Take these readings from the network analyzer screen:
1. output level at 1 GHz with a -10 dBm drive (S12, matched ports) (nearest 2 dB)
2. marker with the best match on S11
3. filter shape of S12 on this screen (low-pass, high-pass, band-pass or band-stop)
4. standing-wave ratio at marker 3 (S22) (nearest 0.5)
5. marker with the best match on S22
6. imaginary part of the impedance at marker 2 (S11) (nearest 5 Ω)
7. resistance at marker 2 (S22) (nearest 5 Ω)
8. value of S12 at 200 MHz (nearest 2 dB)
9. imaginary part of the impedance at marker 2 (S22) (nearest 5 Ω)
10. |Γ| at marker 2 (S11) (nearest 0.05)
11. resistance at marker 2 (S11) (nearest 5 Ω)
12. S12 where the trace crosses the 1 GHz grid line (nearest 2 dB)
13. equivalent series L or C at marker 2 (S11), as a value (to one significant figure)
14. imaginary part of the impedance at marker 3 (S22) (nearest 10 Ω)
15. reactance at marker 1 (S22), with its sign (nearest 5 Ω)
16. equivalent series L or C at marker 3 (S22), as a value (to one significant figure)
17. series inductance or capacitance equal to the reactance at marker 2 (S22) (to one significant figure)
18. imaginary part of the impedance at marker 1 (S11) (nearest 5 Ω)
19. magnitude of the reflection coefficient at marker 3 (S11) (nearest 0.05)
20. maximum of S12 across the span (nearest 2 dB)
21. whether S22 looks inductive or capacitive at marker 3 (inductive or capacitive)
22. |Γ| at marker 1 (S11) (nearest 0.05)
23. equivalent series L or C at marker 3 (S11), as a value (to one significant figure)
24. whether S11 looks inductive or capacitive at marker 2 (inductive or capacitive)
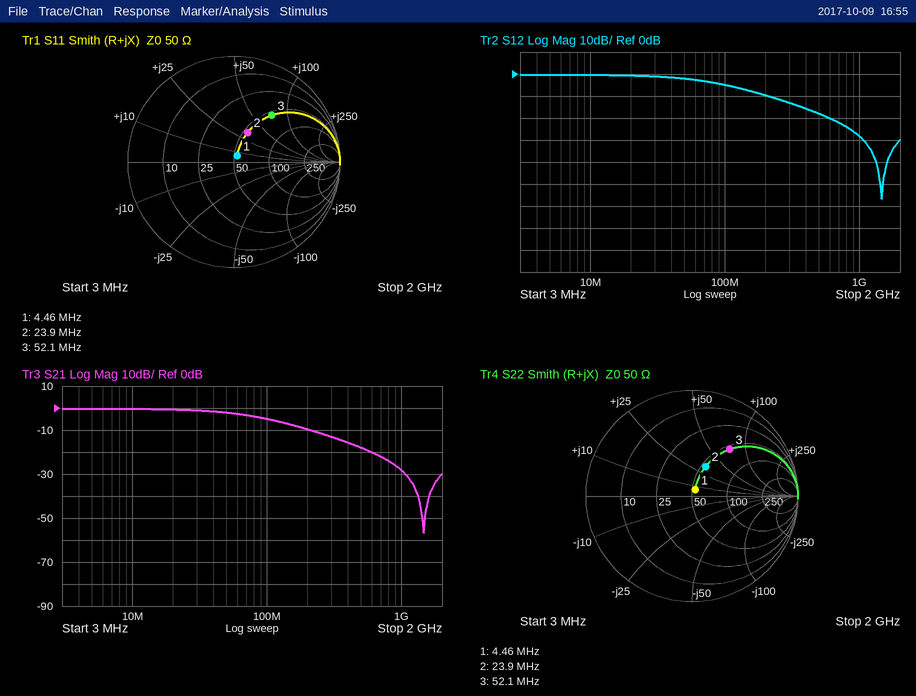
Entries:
-38 dBm
marker 1
low-pass
3.5
marker 1
+35 Ω
55 Ω
-10 dB
+35 Ω
0.30
55 Ω
-28 dB
200 nH
+70 Ω
+5 Ω
200 nH
200 nH
+5 Ω
0.55
0 dB
inductive
0.05
200 nH
inductive
